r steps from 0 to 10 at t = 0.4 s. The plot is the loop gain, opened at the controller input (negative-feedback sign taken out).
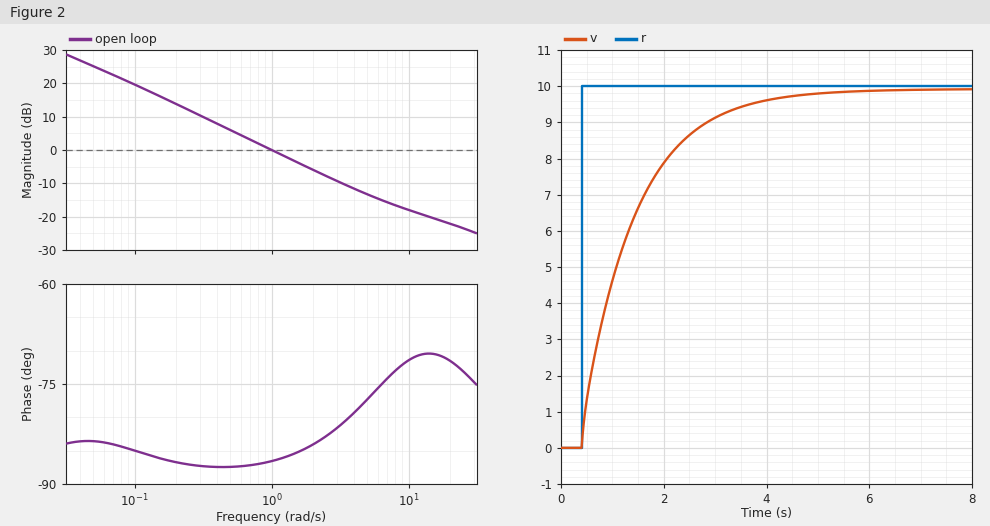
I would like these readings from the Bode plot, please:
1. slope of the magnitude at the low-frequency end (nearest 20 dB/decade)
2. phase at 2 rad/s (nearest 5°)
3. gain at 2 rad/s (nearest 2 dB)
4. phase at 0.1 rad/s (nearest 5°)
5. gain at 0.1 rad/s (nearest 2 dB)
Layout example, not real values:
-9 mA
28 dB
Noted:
-20 dB/decade
-85°
-6 dB
-85°
20 dB
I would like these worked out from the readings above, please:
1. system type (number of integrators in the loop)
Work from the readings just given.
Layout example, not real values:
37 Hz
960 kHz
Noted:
1
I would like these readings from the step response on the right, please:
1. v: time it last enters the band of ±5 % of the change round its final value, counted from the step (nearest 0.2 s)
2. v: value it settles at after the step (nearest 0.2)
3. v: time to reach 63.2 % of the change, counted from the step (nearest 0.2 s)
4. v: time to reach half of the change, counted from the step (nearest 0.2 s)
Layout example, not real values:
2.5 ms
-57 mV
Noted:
3.2 s
10.0
1.0 s
0.6 s
